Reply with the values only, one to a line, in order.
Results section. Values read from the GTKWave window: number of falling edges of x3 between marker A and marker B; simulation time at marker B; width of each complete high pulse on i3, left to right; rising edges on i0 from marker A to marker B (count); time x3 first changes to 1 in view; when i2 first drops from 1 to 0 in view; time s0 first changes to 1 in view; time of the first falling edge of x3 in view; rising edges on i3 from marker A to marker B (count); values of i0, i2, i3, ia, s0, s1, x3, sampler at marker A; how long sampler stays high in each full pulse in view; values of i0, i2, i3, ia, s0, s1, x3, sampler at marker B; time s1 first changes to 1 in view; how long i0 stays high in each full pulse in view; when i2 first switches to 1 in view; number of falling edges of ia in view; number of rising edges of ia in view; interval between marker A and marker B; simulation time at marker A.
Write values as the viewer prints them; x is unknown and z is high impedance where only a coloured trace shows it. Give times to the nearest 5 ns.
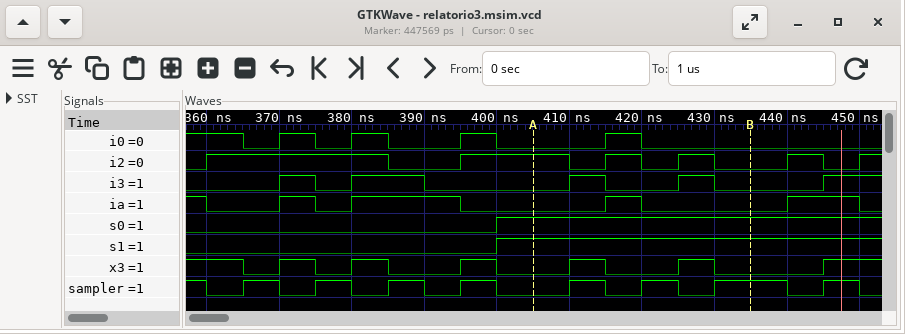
2
435 ns
5 ns, 10 ns, 5 ns, 5 ns
1
370 ns
385 ns
400 ns
365 ns
2
i0=0, i2=1, i3=0, ia=0, s0=1, s1=1, x3=0, sampler=0
5 ns, 5 ns, 5 ns, 5 ns, 5 ns, 5 ns, 10 ns, 5 ns
i0=0, i2=0, i3=0, ia=0, s0=1, s1=1, x3=0, sampler=1
400 ns
5 ns, 5 ns, 5 ns, 5 ns
360 ns
5
4
30 ns
405 ns
